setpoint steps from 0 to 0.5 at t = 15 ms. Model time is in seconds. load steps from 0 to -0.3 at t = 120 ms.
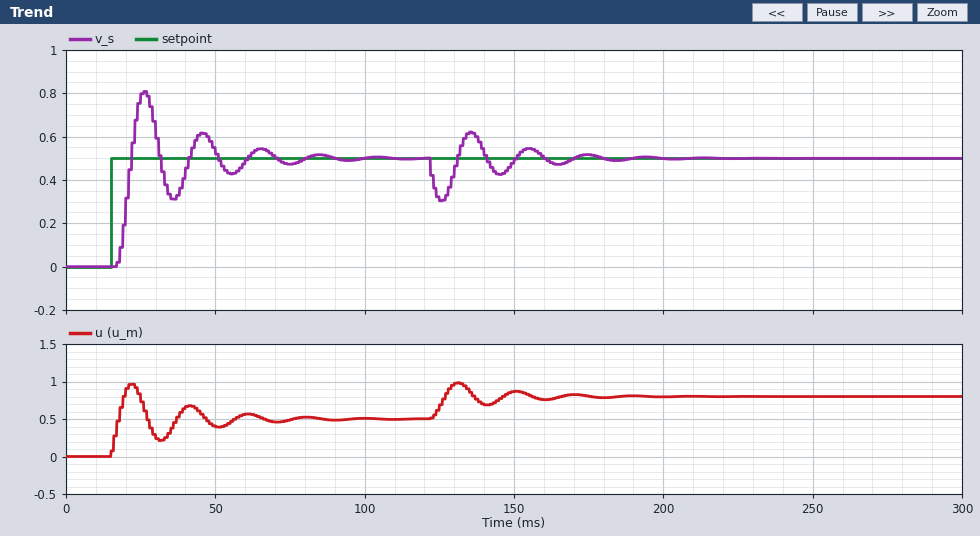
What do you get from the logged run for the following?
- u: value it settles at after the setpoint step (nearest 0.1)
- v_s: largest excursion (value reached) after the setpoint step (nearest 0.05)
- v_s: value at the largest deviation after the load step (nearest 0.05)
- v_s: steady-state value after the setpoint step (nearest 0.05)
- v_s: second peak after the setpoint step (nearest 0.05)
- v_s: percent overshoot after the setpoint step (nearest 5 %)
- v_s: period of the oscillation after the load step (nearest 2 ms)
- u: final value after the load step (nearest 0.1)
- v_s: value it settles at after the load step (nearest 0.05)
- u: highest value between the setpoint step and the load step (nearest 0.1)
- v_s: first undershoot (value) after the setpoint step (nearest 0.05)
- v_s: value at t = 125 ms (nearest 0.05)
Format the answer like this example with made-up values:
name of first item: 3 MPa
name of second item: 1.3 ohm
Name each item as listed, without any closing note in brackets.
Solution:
u: value it settles at after the setpoint step: 0.5
v_s: largest excursion (value reached) after the setpoint step: 0.80
v_s: value at the largest deviation after the load step: 0.30
v_s: steady-state value after the setpoint step: 0.50
v_s: second peak after the setpoint step: 0.60
v_s: percent overshoot after the setpoint step: 60 %
v_s: period of the oscillation after the load step: 20 ms
u: final value after the load step: 0.8
v_s: value it settles at after the load step: 0.50
u: highest value between the setpoint step and the load step: 1.0
v_s: first undershoot (value) after the setpoint step: 0.30
v_s: value at t = 125 ms: 0.30
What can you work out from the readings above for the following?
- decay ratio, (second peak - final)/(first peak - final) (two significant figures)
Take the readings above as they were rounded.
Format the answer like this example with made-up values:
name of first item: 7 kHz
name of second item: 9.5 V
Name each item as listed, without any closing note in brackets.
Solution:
decay ratio, (second peak - final)/(first peak - final): 0.33
